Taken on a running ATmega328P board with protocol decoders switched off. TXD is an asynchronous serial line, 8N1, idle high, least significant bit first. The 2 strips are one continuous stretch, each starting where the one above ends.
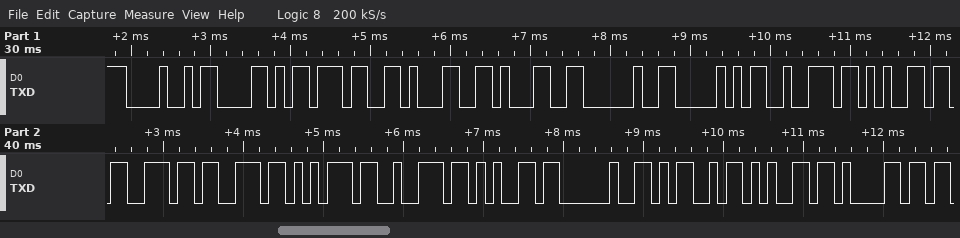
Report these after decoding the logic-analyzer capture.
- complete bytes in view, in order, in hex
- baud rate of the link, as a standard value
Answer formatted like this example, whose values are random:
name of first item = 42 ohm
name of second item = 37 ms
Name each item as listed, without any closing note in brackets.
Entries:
complete bytes in view, in order, in hex = 0x48 0x58 0x37 0x31 0x31 0x20 0x50 0x72 0x65 0x73 0x73 0x75 0x72 0x65 0x20 0x4D 0x65 0x61
baud rate of the link, as a standard value = 9600 baud
